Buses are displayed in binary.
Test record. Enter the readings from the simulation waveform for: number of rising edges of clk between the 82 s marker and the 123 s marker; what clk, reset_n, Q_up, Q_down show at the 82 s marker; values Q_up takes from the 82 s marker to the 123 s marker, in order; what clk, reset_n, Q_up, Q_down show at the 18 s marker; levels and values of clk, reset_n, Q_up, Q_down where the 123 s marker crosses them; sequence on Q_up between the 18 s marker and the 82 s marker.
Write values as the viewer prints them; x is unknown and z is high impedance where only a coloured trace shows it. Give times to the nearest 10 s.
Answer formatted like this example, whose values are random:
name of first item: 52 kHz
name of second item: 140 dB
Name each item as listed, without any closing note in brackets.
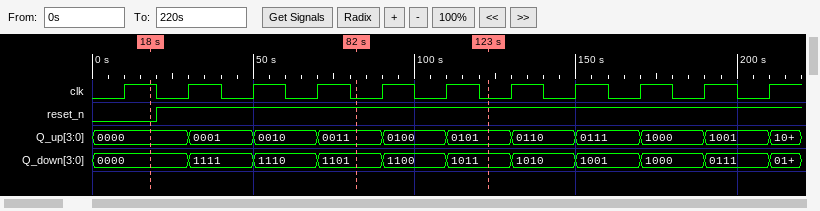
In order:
number of rising edges of clk between the 82 s marker and the 123 s marker: 2
what clk, reset_n, Q_up, Q_down show at the 82 s marker: clk=0, reset_n=1, Q_up=0011, Q_down=1101
values Q_up takes from the 82 s marker to the 123 s marker, in order: 0011, 0100, 0101
what clk, reset_n, Q_up, Q_down show at the 18 s marker: clk=1, reset_n=0, Q_up=0000, Q_down=0000
levels and values of clk, reset_n, Q_up, Q_down where the 123 s marker crosses them: clk=0, reset_n=1, Q_up=0101, Q_down=1011
sequence on Q_up between the 18 s marker and the 82 s marker: 0000, 0001, 0010, 0011
